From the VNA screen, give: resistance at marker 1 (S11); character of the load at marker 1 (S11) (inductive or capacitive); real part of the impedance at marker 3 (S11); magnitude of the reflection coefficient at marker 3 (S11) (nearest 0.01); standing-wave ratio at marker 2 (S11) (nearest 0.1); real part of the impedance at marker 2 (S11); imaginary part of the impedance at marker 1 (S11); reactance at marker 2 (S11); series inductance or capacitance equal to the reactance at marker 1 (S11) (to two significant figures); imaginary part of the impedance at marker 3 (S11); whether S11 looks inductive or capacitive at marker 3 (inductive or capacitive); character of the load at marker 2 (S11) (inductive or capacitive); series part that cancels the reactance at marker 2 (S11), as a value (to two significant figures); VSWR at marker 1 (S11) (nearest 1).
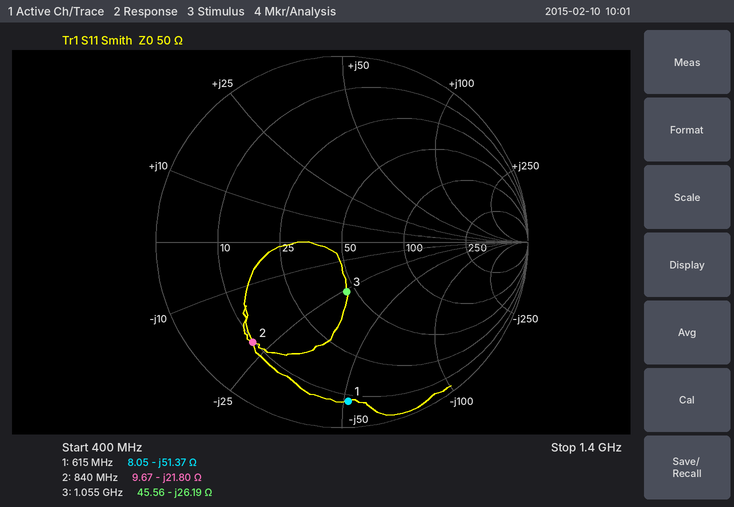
8.05 Ω
capacitive
45.56 Ω
0.27
6.2
9.67 Ω
-51.37 Ω
-21.80 Ω
5.0 pF
-26.19 Ω
capacitive
capacitive
4.1 nH
13
